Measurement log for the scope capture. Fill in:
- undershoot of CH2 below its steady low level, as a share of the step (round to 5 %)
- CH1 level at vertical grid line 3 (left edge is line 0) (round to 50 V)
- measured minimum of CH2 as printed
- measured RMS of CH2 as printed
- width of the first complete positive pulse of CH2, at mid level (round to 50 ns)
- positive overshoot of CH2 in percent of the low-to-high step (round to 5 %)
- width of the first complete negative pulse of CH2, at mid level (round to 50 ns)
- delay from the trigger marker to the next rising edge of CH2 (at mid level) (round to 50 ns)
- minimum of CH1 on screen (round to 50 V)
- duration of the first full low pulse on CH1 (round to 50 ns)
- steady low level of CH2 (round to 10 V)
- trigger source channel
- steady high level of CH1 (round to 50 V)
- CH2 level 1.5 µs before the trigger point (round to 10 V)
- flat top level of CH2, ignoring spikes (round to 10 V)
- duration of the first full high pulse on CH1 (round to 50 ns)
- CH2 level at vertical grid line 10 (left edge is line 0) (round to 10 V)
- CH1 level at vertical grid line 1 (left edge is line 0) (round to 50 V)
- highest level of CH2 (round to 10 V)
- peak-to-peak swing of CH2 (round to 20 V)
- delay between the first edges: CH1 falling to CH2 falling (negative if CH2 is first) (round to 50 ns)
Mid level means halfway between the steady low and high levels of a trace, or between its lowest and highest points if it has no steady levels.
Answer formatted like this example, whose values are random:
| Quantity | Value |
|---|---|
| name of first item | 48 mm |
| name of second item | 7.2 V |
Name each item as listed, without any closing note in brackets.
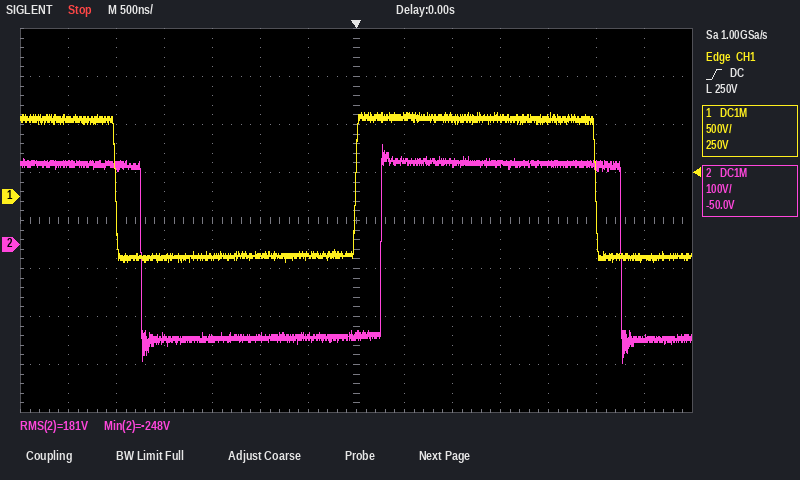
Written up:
| Quantity | Value |
|---|---|
| undershoot of CH2 below its steady low level, as a share of the step | 15 % |
| CH1 level at vertical grid line 3 (left edge is line 0) | -650 V |
| measured minimum of CH2 as printed | -248 V |
| measured RMS of CH2 as printed | 181 V |
| width of the first complete positive pulse of CH2, at mid level | 2.50 µs |
| positive overshoot of CH2 in percent of the low-to-high step | 10 % |
| width of the first complete negative pulse of CH2, at mid level | 2.50 µs |
| delay from the trigger marker to the next rising edge of CH2 (at mid level) | 250 ns |
| minimum of CH1 on screen | -700 V |
| duration of the first full low pulse on CH1 | 2.50 µs |
| steady low level of CH2 | -200 V |
| trigger source channel | CH1 |
| steady high level of CH1 | 800 V |
| CH2 level 1.5 µs before the trigger point | -200 V |
| flat top level of CH2, ignoring spikes | 170 V |
| duration of the first full high pulse on CH1 | 2.50 µs |
| CH2 level at vertical grid line 10 (left edge is line 0) | 170 V |
| CH1 level at vertical grid line 1 (left edge is line 0) | 800 V |
| highest level of CH2 | 210 V |
| peak-to-peak swing of CH2 | 460 V |
| delay between the first edges: CH1 falling to CH2 falling (negative if CH2 is first) | +250 ns |
